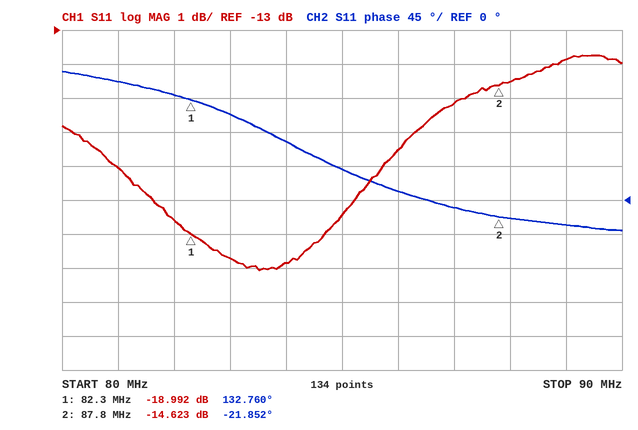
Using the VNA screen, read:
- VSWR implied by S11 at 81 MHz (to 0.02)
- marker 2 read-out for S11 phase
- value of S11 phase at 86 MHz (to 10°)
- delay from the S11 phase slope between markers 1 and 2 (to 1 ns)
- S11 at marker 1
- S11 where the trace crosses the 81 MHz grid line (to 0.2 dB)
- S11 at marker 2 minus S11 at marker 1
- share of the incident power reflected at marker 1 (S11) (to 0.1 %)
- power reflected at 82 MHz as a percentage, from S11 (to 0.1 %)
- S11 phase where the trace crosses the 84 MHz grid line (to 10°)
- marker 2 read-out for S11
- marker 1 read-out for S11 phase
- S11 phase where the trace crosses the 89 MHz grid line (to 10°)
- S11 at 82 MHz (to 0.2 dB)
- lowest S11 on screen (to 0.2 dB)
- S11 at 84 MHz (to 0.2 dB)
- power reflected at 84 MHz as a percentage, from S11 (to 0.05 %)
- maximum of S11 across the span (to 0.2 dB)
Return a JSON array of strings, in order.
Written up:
["1.32", "-21.852°", "10°", "78 ns", "-18.992 dB", "-17.0 dB", "4.369 dB", "1.3 %", "1.4 %", "80°", "-14.623 dB", "132.760°", "-30°", "-18.6 dB", "-20.0 dB", "-19.8 dB", "1.05 %", "-13.8 dB"]
